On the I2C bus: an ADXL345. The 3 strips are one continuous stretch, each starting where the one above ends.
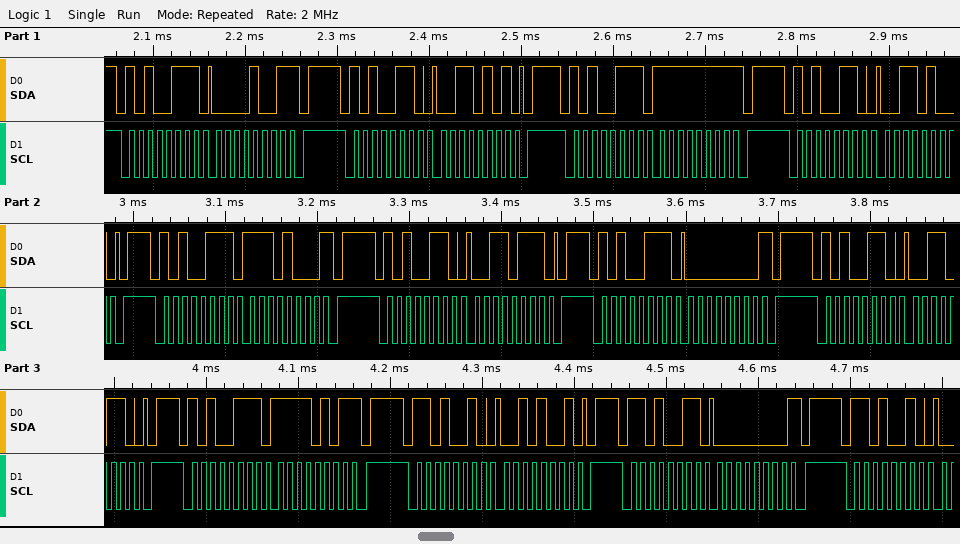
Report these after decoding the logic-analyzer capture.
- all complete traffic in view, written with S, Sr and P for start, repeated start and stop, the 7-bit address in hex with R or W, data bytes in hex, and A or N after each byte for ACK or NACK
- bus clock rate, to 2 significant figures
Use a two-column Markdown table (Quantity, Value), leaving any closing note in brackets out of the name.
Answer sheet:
| Quantity | Value |
|---|---|
| all complete traffic in view, written with S, Sr and P for start, repeated start and stop, the 7-bit address in hex with R or W, data bytes in hex, and A or N after each byte for ACK or NACK | S 53R A 09 N P S 53W A 35 A P S 53R A FF N P S 53W A 34 A P S 53R A E8 N P S 53W A 37 A P S 53R A 00 N P S 53W A 36 A P S 53R A F5 N P S 69W A 29 A P S 69R A 00 N P S 69W A |
| bus clock rate, to 2 significant figures | 100 kHz |
